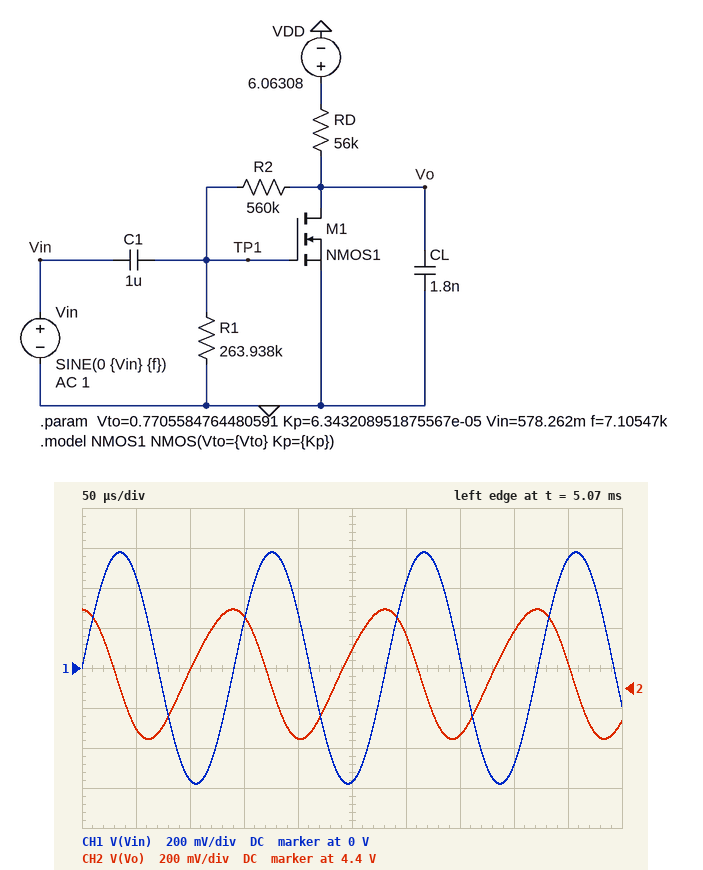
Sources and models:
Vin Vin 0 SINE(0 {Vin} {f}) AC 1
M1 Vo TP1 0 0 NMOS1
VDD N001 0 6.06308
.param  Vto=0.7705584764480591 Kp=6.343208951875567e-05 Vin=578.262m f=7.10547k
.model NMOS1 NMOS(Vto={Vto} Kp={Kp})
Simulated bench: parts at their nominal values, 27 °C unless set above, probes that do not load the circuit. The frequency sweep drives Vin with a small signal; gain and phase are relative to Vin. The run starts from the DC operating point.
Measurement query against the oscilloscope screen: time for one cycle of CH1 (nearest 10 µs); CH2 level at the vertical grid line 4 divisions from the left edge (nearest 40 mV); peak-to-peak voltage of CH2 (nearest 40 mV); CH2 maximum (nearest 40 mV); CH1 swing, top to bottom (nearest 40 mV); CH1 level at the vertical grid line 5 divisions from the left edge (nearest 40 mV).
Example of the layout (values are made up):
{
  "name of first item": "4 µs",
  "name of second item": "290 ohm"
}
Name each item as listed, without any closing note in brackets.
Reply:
{
  "time for one cycle of CH1": "140 µs",
  "CH2 level at the vertical grid line 4 divisions from the left edge": "4.16 V",
  "peak-to-peak voltage of CH2": "640 mV",
  "CH2 maximum": "4.80 V",
  "CH1 swing, top to bottom": "1.16 V",
  "CH1 level at the vertical grid line 5 divisions from the left edge": "-560 mV"
}
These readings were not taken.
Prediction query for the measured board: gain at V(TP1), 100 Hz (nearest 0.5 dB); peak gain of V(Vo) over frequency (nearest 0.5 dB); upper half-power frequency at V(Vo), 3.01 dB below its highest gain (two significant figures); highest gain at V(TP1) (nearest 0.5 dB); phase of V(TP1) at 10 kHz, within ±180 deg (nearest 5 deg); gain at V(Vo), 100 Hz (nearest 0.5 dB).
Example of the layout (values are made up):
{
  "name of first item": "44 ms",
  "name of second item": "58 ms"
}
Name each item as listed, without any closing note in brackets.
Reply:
{
  "gain at V(TP1), 100 Hz": "0 dB",
  "peak gain of V(Vo) over frequency": "7.5 dB",
  "upper half-power frequency at V(Vo), 3.01 dB below its highest gain": "1.7 kHz",
  "highest gain at V(TP1)": "0 dB",
  "phase of V(TP1) at 10 kHz, within ±180 deg": "0 deg",
  "gain at V(Vo), 100 Hz": "7.5 dB"
}
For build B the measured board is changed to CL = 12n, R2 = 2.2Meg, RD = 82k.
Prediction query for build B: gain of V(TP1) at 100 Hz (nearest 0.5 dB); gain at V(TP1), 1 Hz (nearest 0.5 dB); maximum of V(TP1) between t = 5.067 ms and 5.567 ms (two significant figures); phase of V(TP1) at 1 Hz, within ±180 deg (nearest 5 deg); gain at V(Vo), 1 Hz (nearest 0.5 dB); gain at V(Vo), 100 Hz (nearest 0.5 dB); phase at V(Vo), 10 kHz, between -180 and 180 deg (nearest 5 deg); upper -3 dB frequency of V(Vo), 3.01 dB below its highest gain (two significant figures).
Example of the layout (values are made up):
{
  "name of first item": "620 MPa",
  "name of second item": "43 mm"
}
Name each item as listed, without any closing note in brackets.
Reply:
{
  "gain of V(TP1) at 100 Hz": "0 dB",
  "gain at V(TP1), 1 Hz": "-1.5 dB",
  "maximum of V(TP1) between t = 5.067 ms and 5.567 ms": "1.2 V",
  "phase of V(TP1) at 1 Hz, within ±180 deg": "35 deg",
  "gain at V(Vo), 1 Hz": "-30.5 dB",
  "gain at V(Vo), 100 Hz": "-30.0 dB",
  "phase at V(Vo), 10 kHz, between -180 and 180 deg": "-90 deg",
  "upper -3 dB frequency of V(Vo), 3.01 dB below its highest gain": "170 Hz"
}
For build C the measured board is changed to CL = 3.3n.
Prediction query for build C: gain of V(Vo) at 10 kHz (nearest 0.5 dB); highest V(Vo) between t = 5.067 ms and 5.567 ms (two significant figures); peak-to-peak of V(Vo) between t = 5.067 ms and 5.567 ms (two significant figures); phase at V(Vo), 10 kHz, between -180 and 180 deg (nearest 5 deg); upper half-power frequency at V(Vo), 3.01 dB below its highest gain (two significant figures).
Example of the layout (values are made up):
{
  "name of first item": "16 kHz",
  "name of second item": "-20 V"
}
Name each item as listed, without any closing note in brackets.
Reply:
{
  "gain of V(Vo) at 10 kHz": "-13.0 dB",
  "highest V(Vo) between t = 5.067 ms and 5.567 ms": "4.7 V",
  "peak-to-peak of V(Vo) between t = 5.067 ms and 5.567 ms": "360 mV",
  "phase at V(Vo), 10 kHz, between -180 and 180 deg": "95 deg",
  "upper half-power frequency at V(Vo), 3.01 dB below its highest gain": "950 Hz"
}
